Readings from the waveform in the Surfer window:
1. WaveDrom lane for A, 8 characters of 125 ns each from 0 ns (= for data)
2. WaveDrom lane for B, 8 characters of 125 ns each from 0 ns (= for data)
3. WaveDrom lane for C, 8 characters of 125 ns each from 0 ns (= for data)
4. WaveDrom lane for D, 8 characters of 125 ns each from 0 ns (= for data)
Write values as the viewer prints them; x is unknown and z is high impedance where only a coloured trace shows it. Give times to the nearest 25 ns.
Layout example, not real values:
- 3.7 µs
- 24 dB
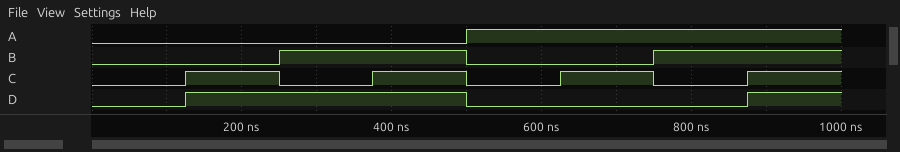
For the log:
- {name: 'A', wave: '0...1...'}
- {name: 'B', wave: '0.1.0.1.'}
- {name: 'C', wave: '01010101'}
- {name: 'D', wave: '01..0..1'}
